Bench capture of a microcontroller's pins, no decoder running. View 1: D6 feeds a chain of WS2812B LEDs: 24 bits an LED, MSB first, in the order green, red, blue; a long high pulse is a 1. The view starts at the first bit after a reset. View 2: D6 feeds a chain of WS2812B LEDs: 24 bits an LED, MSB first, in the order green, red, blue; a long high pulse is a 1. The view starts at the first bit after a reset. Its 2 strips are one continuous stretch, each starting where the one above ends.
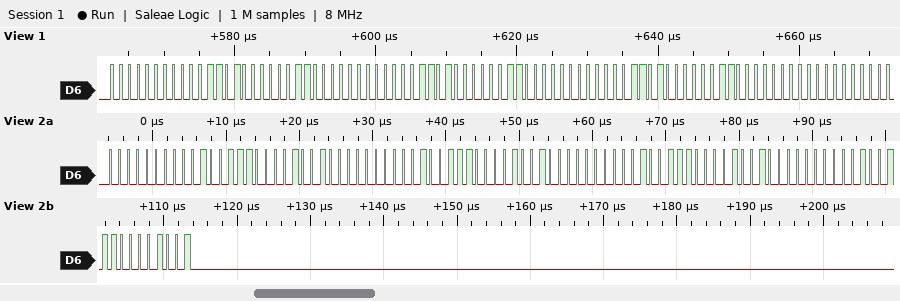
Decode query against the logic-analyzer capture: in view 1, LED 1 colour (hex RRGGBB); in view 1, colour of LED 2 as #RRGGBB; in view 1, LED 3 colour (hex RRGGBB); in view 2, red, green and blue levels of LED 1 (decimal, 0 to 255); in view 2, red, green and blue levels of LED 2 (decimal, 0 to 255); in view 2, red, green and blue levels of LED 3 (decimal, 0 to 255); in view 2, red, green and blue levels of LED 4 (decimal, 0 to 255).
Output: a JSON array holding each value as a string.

["#1A0006", "#1A0006", "#1A0006", "39, 0, 9", "39, 0, 9", "39, 0, 9", "39, 0, 9"]
